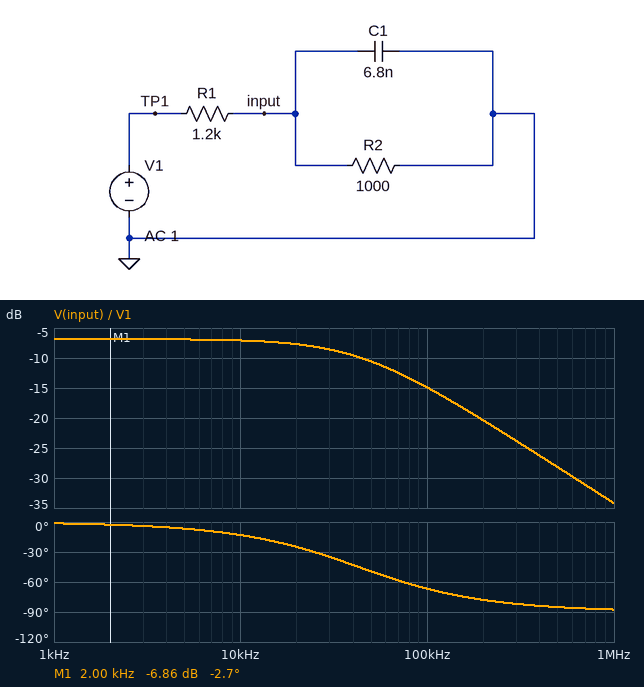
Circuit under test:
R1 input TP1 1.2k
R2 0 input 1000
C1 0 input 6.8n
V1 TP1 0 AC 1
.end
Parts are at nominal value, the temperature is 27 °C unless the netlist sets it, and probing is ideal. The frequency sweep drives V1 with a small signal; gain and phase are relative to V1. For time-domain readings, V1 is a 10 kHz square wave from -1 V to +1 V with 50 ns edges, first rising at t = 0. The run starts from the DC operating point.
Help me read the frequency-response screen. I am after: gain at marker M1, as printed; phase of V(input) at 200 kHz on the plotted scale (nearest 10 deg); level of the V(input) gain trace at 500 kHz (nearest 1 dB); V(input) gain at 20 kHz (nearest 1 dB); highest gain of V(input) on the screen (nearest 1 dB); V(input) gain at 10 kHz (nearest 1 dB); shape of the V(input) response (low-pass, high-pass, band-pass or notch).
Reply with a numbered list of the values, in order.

1. -6.86 dB
2. -80 deg
3. -28 dB
4. -8 dB
5. -7 dB
6. -7 dB
7. low-pass
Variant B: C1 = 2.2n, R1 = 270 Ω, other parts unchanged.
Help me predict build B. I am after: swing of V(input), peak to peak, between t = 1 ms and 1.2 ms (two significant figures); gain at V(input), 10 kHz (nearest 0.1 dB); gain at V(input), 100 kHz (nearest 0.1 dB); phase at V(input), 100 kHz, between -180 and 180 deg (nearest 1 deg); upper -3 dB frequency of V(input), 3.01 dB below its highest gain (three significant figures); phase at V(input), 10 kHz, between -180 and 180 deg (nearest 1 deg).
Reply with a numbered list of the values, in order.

1. 1.6 V
2. -2.1 dB
3. -2.4 dB
4. -16 deg
5. 340 kHz
6. -2 deg
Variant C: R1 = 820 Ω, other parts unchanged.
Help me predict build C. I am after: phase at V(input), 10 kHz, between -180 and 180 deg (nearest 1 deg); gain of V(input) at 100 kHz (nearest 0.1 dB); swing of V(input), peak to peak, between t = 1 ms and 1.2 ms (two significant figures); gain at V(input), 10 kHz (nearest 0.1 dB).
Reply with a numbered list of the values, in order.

1. -11 deg
2. -11.9 dB
3. 1.1 V
4. -5.4 dB
